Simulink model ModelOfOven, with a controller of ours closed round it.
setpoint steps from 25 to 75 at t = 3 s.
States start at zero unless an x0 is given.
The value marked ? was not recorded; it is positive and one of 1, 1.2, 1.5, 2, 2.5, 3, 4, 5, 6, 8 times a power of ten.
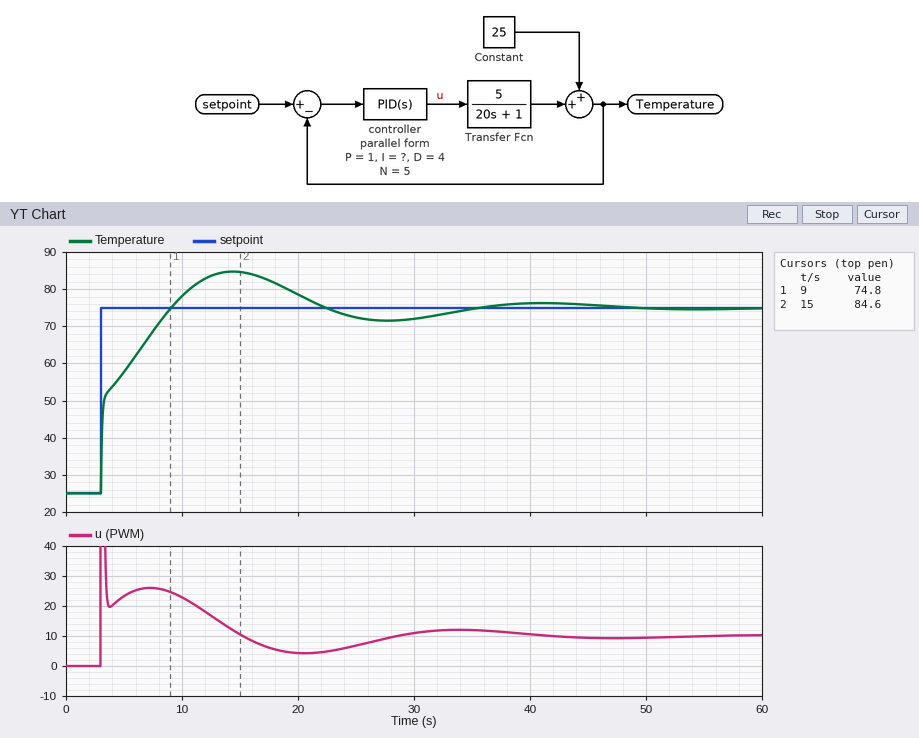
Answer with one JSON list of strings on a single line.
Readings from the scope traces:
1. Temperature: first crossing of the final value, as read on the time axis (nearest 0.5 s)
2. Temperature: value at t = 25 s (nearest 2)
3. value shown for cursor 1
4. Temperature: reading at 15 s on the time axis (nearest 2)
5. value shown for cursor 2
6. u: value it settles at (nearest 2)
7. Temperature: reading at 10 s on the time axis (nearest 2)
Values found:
["9.0 s", "72", "74.8", "84", "84.6", "10", "78"]
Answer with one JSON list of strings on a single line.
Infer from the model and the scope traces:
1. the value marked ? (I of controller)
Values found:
["0.5"]
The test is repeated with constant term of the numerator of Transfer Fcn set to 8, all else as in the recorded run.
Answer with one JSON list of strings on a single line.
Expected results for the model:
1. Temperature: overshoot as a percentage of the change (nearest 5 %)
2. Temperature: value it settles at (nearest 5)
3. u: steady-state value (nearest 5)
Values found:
["15 %", "75", "5"]
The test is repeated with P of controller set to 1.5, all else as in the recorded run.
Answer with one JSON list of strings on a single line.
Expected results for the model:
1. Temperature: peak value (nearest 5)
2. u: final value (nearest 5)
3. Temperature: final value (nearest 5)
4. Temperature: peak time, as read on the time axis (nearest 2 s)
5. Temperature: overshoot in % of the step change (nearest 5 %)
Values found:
["80", "10", "75", "14 s", "15 %"]
